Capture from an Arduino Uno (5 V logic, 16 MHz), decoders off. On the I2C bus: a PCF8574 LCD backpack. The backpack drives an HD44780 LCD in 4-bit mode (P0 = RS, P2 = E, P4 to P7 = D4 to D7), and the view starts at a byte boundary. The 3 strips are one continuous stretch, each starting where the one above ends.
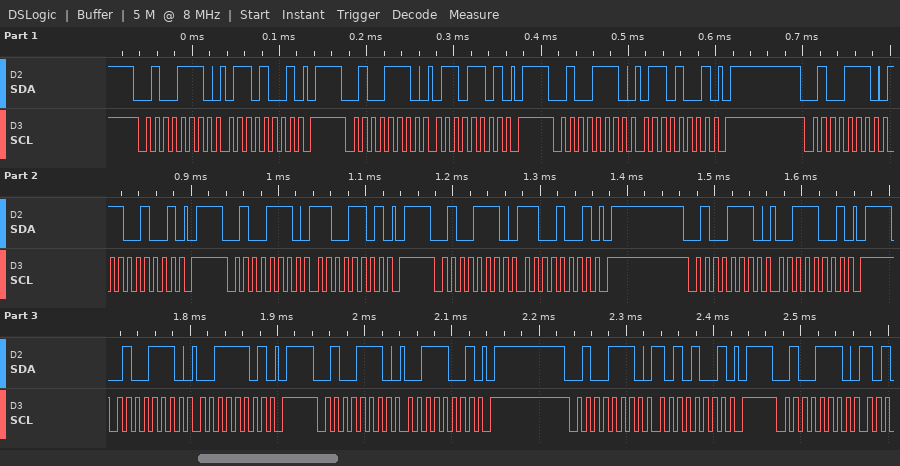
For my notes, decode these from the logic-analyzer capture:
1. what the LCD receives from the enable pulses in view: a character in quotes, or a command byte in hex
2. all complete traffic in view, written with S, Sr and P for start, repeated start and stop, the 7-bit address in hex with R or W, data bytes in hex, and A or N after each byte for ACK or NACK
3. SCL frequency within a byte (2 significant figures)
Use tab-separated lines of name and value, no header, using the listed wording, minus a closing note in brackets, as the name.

what the LCD receives from the enable pulses in view: a character in quotes, or a command byte in hex	'l'
all complete traffic in view, written with S, Sr and P for start, repeated start and stop, the 7-bit address in hex with R or W, data bytes in hex, and A or N after each byte for ACK or NACK	S 27W A 69 A P S 27W A 6D A P S 27W A 69 A P S 27W A C9 A P S 27W A CD A P S 27W A C9 A P S 27W A 39 A P S 27W A 3D A P S 27W A 39 A P S 27W A A9 A P S 27W A
SCL frequency within a byte	100 kHz
